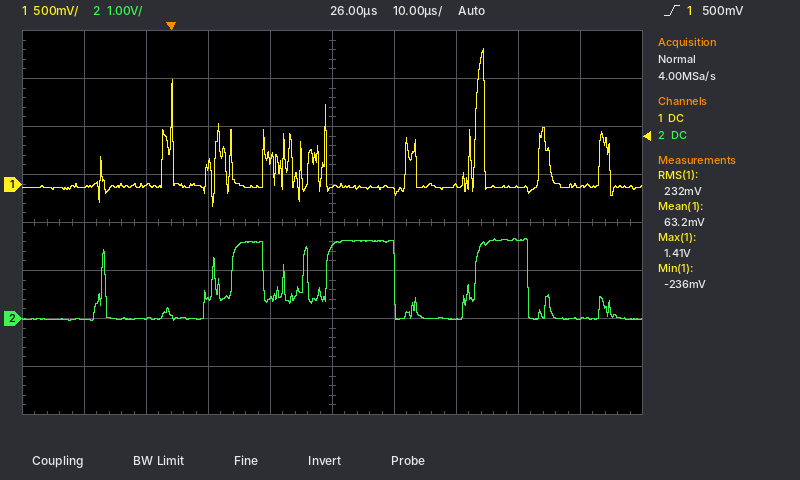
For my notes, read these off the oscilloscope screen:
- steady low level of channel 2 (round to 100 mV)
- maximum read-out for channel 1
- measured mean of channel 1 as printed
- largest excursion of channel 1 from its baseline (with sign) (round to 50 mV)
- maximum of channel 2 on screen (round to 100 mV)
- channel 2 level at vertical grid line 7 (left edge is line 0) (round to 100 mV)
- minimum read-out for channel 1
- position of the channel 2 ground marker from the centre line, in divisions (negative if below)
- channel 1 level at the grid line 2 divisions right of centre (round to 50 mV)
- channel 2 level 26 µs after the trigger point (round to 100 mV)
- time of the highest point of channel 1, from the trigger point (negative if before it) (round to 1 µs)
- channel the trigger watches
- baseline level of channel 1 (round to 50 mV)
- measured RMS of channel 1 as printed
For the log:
0.0 V
1.41 V
63.2 mV
+1.45 V
1.7 V
0.0 V
-236 mV
-2.0 div
0 mV
1.5 V
+50 µs
channel 1
-50 mV
232 mV
